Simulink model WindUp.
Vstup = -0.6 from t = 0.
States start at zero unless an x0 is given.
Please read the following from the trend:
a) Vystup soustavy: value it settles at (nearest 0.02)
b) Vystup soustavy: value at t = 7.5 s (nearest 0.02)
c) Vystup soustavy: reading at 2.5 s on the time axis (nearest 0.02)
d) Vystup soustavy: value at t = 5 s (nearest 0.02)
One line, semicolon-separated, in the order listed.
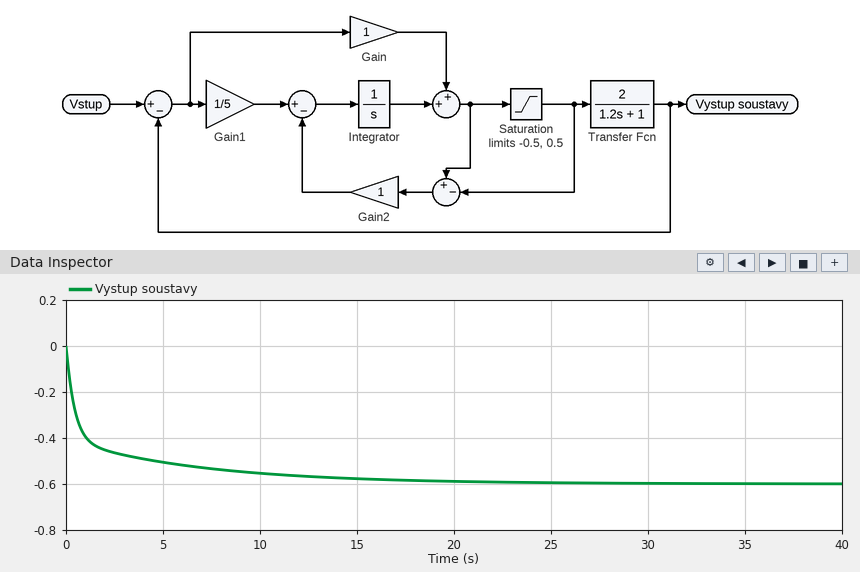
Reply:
-0.60; -0.54; -0.46; -0.50
